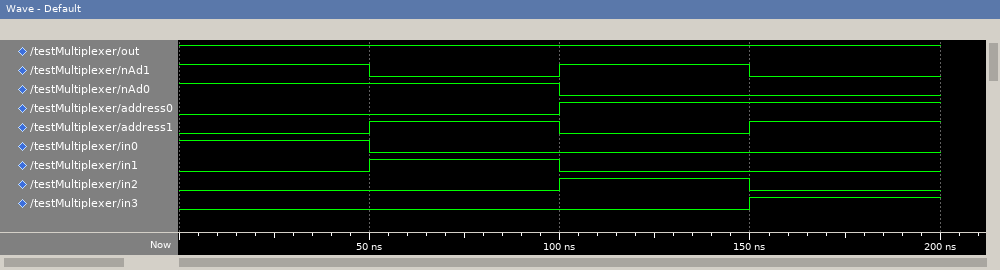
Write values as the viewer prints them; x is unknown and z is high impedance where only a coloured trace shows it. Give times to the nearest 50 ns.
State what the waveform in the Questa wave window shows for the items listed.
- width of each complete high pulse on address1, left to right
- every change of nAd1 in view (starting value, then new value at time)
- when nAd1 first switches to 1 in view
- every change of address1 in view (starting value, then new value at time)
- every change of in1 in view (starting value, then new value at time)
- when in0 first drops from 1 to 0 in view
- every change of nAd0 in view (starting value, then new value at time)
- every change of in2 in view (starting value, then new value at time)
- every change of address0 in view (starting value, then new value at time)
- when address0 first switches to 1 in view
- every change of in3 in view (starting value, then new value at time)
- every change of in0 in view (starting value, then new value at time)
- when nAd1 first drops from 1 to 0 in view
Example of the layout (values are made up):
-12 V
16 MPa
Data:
50 ns
1, 0 at 50 ns, 1 at 100 ns, 0 at 150 ns
100 ns
0, 1 at 50 ns, 0 at 100 ns, 1 at 150 ns
0, 1 at 50 ns, 0 at 100 ns
50 ns
1, 0 at 100 ns
0, 1 at 100 ns, 0 at 150 ns
0, 1 at 100 ns
100 ns
0, 1 at 150 ns
1, 0 at 50 ns
50 ns
